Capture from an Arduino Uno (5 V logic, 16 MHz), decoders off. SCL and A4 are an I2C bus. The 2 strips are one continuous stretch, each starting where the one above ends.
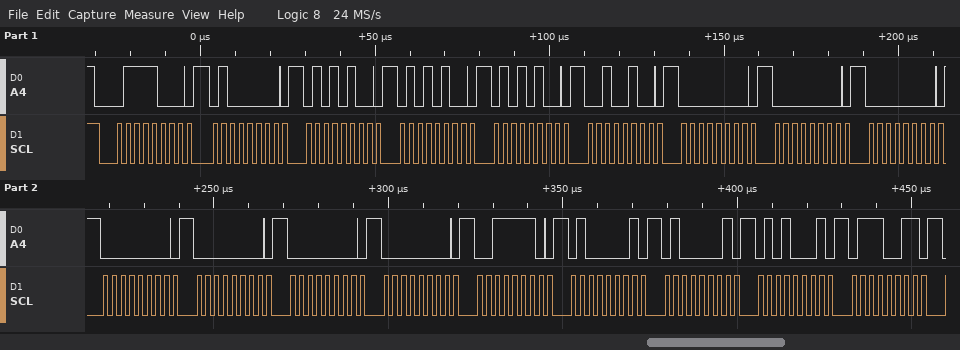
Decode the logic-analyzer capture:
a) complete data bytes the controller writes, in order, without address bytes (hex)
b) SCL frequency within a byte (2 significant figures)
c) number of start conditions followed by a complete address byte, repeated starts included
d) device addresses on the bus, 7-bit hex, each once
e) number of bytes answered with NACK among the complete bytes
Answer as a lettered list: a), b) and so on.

a) 40 54 54 54 24 00 00 00 00 00 00 00 3E 41 41 51 73
b) 400 kHz
c) 1
d) 0x3C
e) 0
